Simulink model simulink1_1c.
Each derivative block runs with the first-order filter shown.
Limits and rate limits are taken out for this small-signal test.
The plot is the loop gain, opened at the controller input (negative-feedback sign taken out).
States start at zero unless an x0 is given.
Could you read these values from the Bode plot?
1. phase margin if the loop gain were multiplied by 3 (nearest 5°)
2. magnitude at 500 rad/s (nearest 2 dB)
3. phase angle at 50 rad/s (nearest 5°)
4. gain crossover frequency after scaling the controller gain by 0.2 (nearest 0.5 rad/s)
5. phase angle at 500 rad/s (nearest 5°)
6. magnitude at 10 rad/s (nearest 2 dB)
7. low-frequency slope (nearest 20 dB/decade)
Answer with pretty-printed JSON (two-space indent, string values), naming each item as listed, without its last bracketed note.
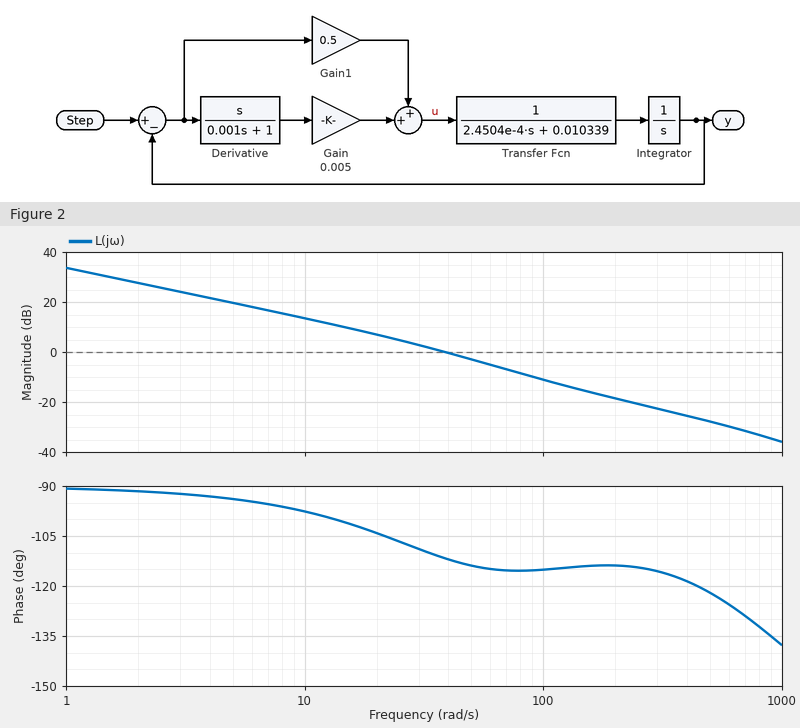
{
  "phase margin if the loop gain were multiplied by 3": "65°",
  "magnitude at 500 rad/s": "-28 dB",
  "phase angle at 50 rad/s": "-115°",
  "gain crossover frequency after scaling the controller gain by 0.2": "9.5 rad/s",
  "phase angle at 500 rad/s": "-120°",
  "magnitude at 10 rad/s": "14 dB",
  "low-frequency slope": "-20 dB/decade"
}
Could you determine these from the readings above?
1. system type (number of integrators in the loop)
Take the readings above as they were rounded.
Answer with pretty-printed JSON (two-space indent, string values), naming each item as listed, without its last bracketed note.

{
  "system type": "1"
}
